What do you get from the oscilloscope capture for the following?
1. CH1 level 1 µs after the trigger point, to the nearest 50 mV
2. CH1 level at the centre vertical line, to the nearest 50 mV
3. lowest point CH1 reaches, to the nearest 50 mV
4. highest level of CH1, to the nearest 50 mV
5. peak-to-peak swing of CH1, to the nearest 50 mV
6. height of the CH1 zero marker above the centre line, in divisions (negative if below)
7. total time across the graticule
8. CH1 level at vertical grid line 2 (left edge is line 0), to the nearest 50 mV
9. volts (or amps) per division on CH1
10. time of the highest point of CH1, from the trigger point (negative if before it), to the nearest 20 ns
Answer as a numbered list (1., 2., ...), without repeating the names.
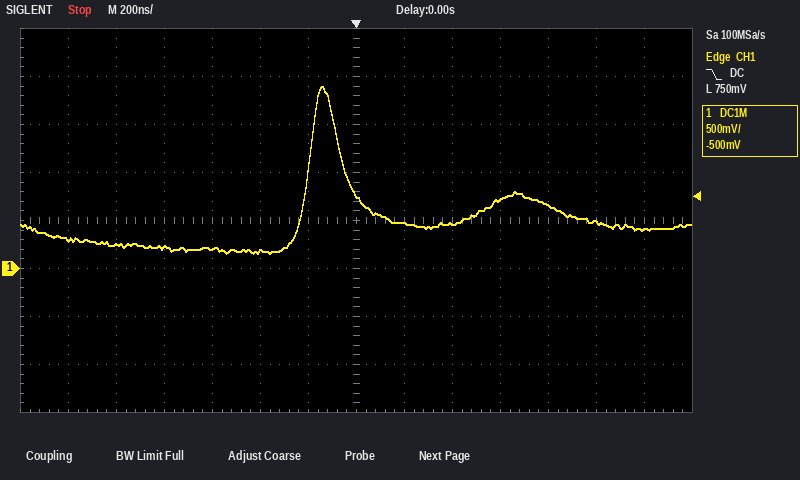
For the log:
1. 500 mV
2. 750 mV
3. 150 mV
4. 1.90 V
5. 1.75 V
6. -1.0 div
7. 2.8 µs
8. 250 mV
9. 500 mV
10. -140 ns
